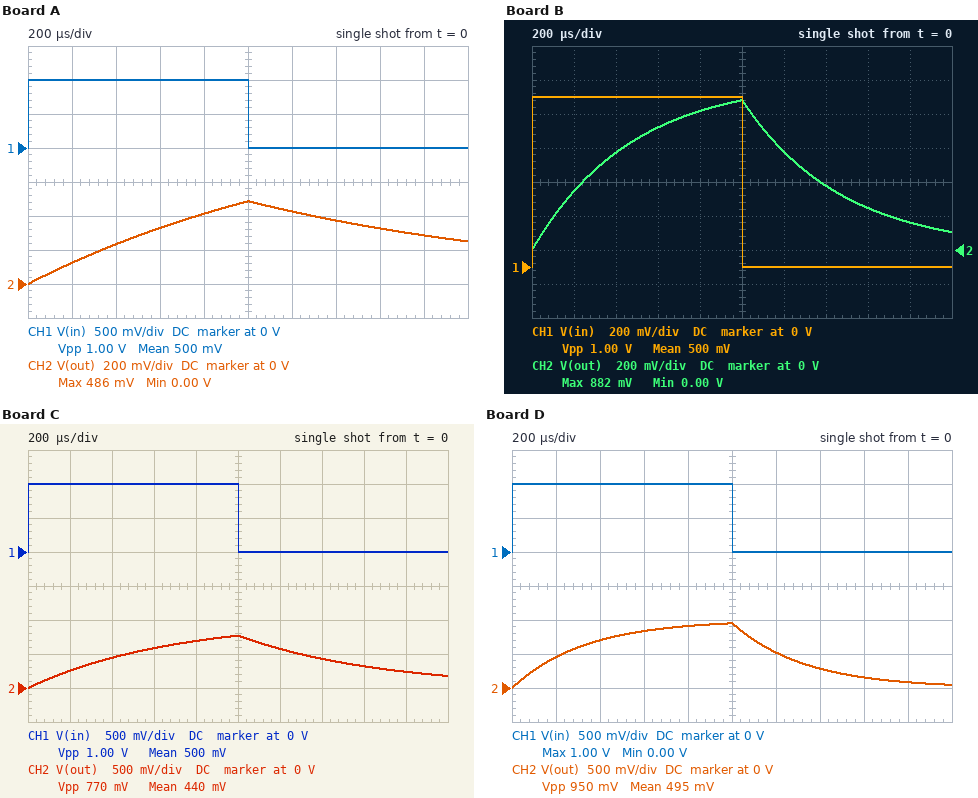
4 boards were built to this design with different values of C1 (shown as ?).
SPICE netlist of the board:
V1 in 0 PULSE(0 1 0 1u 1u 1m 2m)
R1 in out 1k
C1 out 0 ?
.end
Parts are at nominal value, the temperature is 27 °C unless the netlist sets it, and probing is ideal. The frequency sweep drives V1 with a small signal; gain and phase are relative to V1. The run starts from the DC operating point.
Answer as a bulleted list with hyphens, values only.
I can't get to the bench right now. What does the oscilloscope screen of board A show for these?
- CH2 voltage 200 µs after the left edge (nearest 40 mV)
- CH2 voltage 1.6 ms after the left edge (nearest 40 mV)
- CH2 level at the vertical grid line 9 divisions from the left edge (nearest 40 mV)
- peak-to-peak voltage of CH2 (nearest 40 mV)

- 120 mV
- 320 mV
- 280 mV
- 480 mV
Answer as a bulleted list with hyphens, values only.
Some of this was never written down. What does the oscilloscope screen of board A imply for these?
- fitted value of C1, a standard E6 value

- 1.5 µF
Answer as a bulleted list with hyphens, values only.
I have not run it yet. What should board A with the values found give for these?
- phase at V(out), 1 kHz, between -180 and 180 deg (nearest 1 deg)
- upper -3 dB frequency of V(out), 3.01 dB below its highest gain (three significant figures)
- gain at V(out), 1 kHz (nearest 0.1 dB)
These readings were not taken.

- -84 deg
- 106 Hz
- -19.5 dB
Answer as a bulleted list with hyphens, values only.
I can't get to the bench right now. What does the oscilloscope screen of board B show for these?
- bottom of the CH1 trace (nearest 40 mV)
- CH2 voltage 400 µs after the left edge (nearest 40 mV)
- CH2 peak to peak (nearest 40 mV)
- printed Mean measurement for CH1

- 0 V
- 560 mV
- 880 mV
- 500 mV
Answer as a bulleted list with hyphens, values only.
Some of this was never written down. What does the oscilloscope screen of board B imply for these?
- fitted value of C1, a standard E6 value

- 470 nF
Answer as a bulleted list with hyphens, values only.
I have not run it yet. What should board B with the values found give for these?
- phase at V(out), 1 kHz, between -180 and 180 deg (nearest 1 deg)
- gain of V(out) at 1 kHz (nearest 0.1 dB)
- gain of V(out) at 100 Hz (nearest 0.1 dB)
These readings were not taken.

- -71 deg
- -9.9 dB
- -0.4 dB
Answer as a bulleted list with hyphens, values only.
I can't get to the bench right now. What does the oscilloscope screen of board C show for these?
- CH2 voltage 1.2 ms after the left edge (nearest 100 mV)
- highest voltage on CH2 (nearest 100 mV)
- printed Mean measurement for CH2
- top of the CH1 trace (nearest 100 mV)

- 600 mV
- 800 mV
- 440 mV
- 1.0 V
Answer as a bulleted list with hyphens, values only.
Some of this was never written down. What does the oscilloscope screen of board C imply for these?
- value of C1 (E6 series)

- 680 nF
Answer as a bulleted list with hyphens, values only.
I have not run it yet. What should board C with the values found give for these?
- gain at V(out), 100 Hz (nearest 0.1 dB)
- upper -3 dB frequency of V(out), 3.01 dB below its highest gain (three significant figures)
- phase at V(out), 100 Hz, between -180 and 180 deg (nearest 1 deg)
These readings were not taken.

- -0.7 dB
- 234 Hz
- -23 deg
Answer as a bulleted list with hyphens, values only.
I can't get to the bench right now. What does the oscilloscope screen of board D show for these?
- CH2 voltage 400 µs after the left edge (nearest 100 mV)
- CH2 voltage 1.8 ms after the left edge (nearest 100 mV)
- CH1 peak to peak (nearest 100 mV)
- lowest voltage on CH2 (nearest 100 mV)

- 700 mV
- 100 mV
- 1.0 V
- 0 V
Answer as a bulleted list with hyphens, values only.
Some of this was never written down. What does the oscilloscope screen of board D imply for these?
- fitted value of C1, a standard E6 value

- 330 nF
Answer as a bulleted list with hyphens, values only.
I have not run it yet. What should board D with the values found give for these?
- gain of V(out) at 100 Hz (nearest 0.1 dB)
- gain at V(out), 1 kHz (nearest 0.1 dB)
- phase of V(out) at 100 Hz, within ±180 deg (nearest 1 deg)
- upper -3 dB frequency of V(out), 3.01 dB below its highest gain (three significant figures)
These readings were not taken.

- -0.2 dB
- -7.2 dB
- -12 deg
- 482 Hz
